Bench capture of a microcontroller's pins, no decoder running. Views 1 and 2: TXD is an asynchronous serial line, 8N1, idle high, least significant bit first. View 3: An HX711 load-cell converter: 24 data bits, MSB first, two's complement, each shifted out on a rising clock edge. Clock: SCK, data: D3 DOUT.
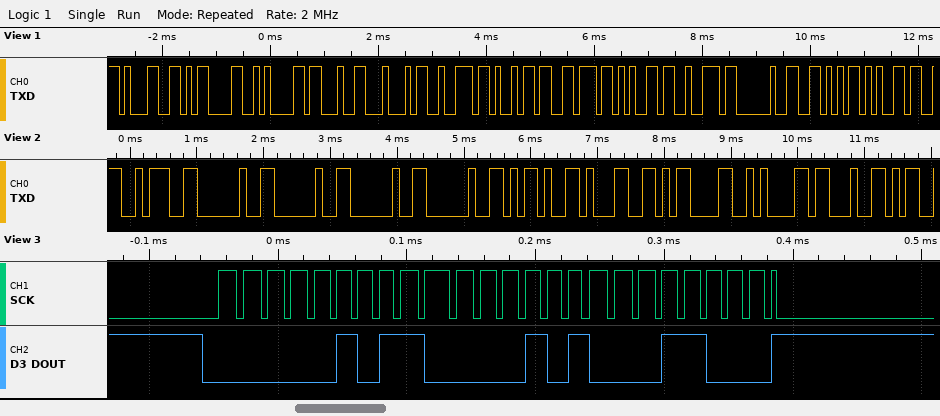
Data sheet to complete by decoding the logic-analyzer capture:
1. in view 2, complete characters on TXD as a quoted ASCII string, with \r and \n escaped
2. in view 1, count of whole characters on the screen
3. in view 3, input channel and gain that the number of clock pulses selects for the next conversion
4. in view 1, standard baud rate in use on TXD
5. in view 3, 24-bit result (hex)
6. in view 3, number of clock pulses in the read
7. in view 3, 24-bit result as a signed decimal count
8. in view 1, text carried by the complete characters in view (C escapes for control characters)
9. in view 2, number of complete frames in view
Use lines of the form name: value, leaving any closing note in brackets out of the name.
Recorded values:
in view 2, complete characters on TXD as a quoted ASCII string, with \r and \n escaped: ":    -1\r\n#"
in view 1, count of whole characters on the screen: 13
in view 3, input channel and gain that the number of clock pulses selects for the next conversion: channel A, gain 128
in view 1, standard baud rate in use on TXD: 9600 baud
in view 3, 24-bit result: 0x058518
in view 3, number of clock pulses in the read: 25
in view 3, 24-bit result as a signed decimal count: 361752
in view 1, text carried by the complete characters in view: "1\r\n#Driver Ve"
in view 2, number of complete frames in view: 10
